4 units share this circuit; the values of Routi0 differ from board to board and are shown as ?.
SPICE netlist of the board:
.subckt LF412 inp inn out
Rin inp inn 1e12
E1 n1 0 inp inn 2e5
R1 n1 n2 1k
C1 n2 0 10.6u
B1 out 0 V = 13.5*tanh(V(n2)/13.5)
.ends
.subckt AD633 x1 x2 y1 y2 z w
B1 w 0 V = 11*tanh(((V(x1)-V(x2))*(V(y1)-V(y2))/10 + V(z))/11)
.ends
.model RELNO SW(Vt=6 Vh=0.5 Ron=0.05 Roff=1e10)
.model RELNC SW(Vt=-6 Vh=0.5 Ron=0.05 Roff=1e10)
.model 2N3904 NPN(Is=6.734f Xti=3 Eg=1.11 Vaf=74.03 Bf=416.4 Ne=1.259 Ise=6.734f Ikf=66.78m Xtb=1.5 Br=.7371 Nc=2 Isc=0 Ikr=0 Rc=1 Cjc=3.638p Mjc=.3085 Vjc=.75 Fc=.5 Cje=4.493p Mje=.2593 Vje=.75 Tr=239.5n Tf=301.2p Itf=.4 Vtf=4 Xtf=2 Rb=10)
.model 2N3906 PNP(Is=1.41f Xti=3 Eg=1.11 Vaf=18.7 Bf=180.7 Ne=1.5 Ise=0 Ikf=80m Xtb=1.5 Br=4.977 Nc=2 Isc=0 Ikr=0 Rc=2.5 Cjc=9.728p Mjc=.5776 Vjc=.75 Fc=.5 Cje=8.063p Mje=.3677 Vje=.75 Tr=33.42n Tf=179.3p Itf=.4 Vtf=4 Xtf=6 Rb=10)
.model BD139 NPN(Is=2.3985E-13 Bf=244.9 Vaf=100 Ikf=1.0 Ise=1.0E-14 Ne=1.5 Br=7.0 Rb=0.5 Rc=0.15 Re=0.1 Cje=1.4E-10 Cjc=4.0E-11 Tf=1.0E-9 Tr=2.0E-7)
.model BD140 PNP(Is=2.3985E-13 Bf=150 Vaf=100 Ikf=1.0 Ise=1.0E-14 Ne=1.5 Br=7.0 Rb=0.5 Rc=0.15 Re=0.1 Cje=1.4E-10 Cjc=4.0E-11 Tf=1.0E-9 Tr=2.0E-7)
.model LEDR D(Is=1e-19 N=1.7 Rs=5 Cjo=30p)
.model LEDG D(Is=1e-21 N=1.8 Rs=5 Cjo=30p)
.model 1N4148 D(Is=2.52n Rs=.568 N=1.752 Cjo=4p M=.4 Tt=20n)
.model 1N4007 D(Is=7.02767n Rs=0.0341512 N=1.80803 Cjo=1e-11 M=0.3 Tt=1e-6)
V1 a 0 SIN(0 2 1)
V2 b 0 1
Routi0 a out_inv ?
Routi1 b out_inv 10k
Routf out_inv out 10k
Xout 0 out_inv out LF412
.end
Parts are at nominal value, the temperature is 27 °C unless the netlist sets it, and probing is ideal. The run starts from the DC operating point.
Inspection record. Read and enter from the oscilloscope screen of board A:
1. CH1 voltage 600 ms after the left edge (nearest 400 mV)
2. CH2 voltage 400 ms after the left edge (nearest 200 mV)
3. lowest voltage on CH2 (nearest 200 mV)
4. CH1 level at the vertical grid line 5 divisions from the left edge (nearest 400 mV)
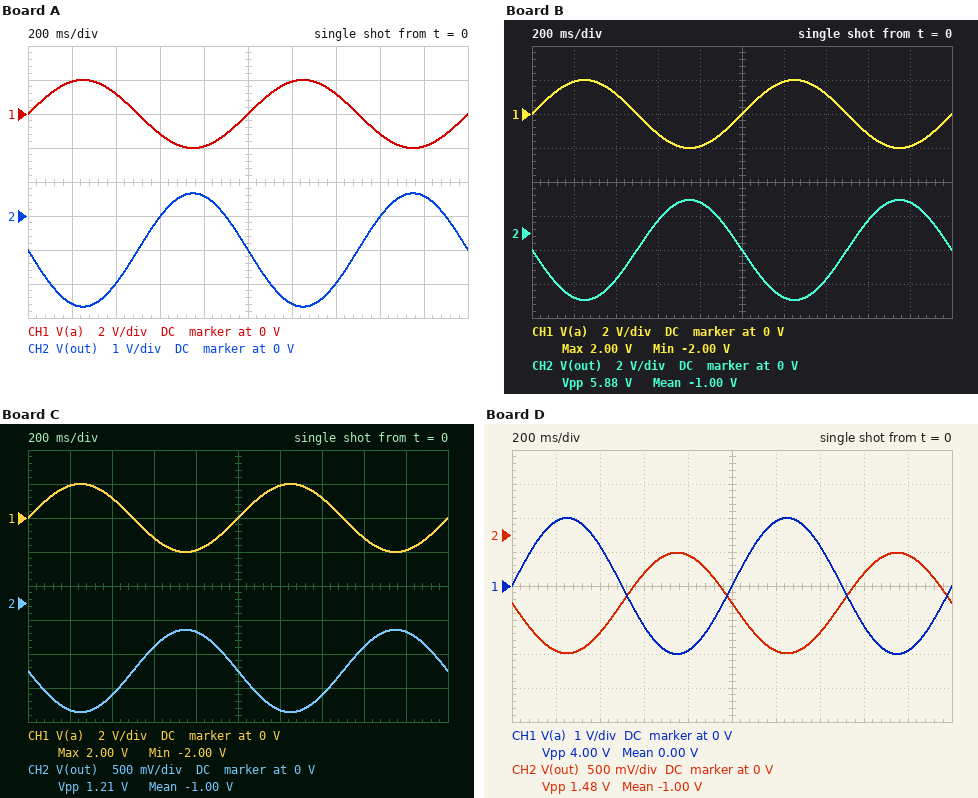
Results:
-1.2 V
-2.0 V
-2.6 V
0 V
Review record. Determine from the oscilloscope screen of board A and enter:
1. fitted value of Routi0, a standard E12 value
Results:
12 kΩ
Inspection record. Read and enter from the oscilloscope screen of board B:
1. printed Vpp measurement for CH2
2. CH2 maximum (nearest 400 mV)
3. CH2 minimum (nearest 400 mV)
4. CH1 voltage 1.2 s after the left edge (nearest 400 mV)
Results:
5.88 V
2.0 V
-4.0 V
2.0 V
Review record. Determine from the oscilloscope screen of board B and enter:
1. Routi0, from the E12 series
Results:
6.8 kΩ
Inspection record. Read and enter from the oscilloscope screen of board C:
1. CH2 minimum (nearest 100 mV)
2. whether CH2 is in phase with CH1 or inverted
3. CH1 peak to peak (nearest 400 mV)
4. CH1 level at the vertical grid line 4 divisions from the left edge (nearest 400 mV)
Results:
-1.6 V
inverted
4.0 V
-2.0 V
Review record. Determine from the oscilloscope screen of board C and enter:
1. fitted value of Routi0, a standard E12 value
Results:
33 kΩ
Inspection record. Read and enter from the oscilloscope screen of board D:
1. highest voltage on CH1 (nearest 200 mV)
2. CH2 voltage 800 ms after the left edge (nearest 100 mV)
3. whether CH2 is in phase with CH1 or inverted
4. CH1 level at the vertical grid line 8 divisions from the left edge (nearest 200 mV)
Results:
2.0 V
-300 mV
inverted
-1.2 V
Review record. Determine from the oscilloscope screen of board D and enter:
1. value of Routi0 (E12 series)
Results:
27 kΩ
